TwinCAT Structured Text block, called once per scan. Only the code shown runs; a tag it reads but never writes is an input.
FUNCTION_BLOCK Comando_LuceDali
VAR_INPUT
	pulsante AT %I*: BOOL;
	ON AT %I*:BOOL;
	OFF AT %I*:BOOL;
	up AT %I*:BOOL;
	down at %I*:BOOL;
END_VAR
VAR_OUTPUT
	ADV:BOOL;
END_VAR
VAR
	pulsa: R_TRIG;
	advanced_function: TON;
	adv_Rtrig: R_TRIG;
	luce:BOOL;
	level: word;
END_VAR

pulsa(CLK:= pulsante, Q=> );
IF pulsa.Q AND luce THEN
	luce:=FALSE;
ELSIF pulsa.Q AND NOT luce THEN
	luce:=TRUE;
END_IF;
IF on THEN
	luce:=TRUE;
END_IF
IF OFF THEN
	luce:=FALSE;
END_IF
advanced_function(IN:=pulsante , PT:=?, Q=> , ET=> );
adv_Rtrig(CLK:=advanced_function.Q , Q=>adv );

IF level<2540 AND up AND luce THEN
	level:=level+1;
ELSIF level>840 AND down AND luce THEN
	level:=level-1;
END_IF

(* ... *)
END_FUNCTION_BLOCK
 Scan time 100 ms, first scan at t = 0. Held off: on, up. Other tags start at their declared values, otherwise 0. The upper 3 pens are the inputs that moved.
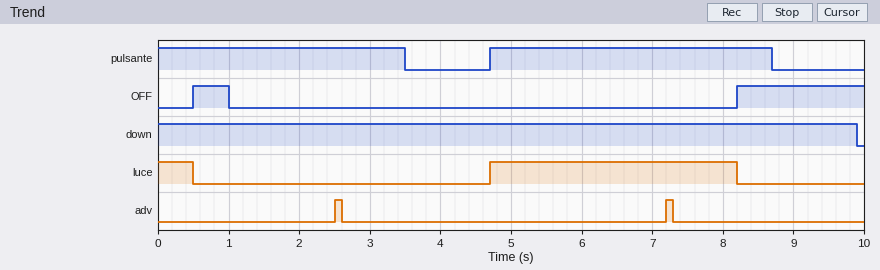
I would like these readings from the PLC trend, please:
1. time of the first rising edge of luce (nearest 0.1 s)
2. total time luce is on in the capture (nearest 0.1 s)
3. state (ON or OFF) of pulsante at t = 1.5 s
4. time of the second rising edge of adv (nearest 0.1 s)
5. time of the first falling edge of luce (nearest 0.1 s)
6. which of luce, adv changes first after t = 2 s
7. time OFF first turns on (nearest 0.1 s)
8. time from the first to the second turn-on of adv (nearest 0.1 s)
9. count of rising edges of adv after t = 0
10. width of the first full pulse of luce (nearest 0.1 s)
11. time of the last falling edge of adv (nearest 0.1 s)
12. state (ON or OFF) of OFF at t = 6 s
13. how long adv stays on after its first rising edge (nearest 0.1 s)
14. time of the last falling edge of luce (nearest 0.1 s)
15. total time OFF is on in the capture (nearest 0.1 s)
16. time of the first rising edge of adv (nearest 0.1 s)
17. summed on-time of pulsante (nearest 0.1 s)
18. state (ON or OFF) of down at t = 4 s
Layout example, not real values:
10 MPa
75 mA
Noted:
4.7 s
4.0 s
ON
7.2 s
0.5 s
adv
0.5 s
4.7 s
2
3.5 s
7.3 s
OFF
0.1 s
8.2 s
2.3 s
2.5 s
7.5 s
ON
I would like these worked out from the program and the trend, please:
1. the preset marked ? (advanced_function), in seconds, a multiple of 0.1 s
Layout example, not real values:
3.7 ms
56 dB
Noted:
2.5 s
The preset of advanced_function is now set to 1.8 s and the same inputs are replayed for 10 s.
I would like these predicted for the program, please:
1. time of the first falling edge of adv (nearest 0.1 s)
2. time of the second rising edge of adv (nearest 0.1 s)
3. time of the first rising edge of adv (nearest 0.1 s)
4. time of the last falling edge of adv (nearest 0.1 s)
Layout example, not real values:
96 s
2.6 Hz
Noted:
1.9 s
6.5 s
1.8 s
6.6 s
